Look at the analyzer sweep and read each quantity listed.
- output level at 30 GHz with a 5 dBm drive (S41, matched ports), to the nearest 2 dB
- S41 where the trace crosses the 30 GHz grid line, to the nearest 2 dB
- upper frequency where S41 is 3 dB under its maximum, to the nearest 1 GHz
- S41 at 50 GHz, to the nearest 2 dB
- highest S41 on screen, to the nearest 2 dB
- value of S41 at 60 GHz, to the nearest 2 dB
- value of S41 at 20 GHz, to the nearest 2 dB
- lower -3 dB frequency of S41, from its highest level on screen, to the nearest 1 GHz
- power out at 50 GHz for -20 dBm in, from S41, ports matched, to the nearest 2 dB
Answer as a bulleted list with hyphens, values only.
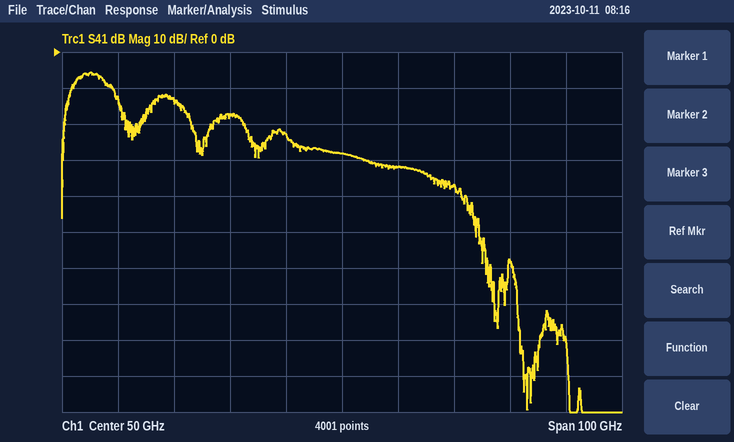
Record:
- -12 dBm
- -18 dB
- 8 GHz
- -28 dB
- -6 dB
- -32 dB
- -14 dB
- 2 GHz
- -48 dBm
